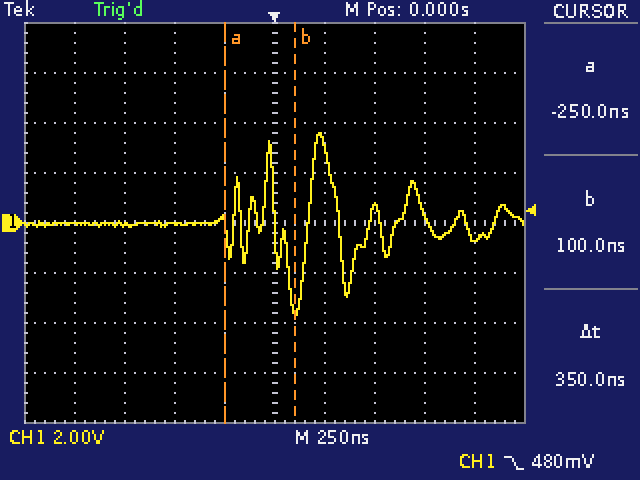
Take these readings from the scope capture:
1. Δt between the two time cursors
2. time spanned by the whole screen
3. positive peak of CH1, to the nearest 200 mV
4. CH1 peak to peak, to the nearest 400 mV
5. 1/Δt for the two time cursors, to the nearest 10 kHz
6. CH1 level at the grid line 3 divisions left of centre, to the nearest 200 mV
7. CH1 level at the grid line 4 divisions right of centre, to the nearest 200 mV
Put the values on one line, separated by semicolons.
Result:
350 ns; 2.5 µs; 3.6 V; 7.2 V; 2.86 MHz; 0.0 V; -600 mV
